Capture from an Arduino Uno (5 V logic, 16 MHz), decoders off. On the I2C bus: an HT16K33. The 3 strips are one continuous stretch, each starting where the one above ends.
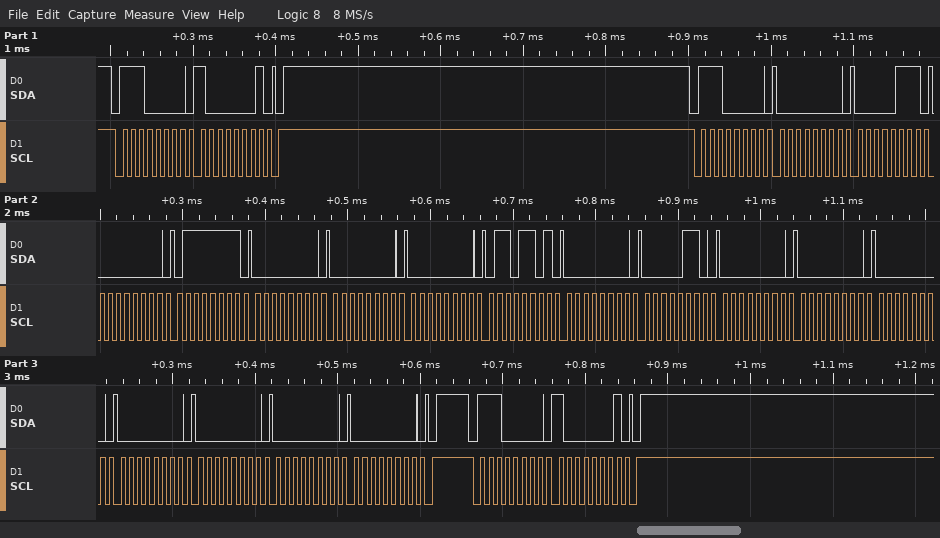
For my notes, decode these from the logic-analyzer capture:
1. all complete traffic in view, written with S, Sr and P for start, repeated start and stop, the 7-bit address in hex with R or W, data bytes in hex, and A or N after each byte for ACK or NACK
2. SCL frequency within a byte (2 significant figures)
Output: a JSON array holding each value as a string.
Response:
["S 70W A 81 A P S 70W A 00 A 07 A 00 A 7F A 00 A 00 A 00 A 6D A 00 A 06 A 00 A 00 A 00 A 00 A 00 A 00 A 00 A P S 70W A 81 A P", "100 kHz"]
